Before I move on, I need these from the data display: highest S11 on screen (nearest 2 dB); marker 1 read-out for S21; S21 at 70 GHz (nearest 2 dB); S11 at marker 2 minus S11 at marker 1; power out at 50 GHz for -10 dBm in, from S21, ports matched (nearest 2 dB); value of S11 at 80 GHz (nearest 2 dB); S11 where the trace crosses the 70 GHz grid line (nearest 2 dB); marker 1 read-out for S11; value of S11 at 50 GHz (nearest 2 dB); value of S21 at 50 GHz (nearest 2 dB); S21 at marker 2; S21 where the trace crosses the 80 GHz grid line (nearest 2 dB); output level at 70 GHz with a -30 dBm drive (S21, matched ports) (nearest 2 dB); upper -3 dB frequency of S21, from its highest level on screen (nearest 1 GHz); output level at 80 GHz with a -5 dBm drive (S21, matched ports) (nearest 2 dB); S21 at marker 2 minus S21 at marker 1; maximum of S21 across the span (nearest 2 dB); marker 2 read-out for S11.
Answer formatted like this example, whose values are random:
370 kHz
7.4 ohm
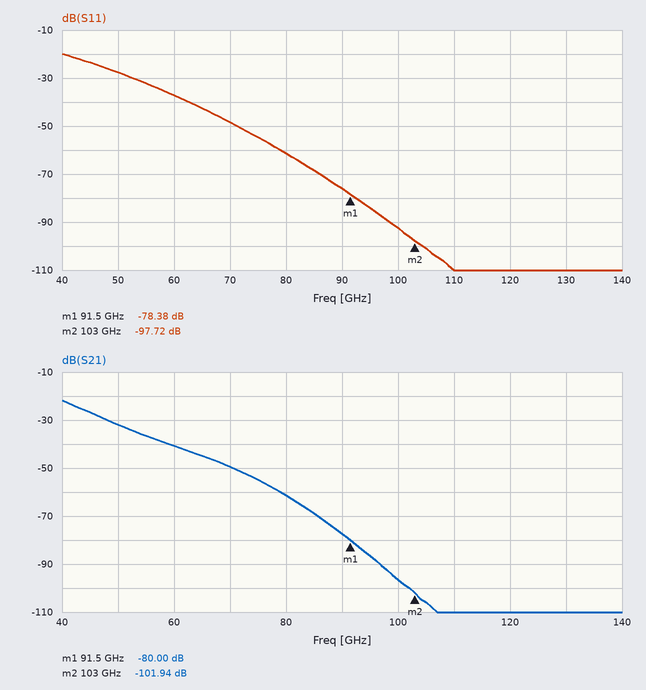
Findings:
-20 dB
-80.00 dB
-50 dB
-19.34 dB
-42 dBm
-62 dB
-48 dB
-78.38 dB
-28 dB
-32 dB
-101.94 dB
-62 dB
-80 dBm
43 GHz
-66 dBm
-21.94 dB
-22 dB
-97.72 dB
